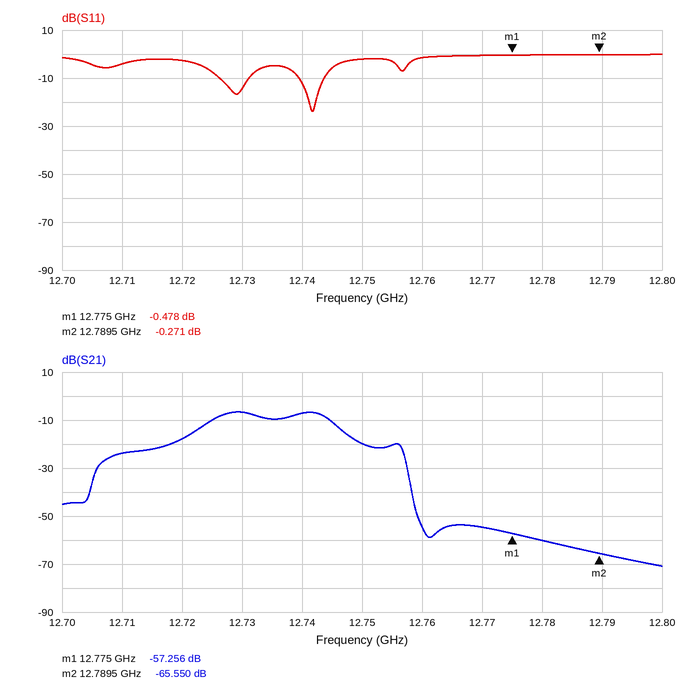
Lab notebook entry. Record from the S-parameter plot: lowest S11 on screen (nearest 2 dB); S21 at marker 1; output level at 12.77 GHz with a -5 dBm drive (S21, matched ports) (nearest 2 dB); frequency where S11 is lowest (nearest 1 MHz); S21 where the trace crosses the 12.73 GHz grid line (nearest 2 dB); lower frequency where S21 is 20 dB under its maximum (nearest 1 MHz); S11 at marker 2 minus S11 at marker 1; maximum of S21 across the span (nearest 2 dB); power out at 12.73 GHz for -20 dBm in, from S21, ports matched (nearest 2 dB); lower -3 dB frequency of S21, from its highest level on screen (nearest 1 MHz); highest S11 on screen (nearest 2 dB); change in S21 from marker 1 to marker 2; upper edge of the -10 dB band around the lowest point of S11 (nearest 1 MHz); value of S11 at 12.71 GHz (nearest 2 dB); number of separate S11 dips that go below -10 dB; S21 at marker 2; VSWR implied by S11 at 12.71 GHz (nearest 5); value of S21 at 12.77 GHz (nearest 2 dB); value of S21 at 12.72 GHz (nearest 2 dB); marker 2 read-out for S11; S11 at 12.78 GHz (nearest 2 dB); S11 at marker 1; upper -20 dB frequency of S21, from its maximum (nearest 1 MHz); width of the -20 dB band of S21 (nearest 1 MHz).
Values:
-24 dB
-57.256 dB
-60 dBm
12.742 GHz
-6 dB
12.707 GHz
0.207 dB
-6 dB
-26 dBm
12.725 GHz
0 dB
-8.294 dB
12.744 GHz
-4 dB
2
-65.550 dB
5
-54 dB
-18 dB
-0.271 dB
0 dB
-0.478 dB
12.757 GHz
50 MHz
